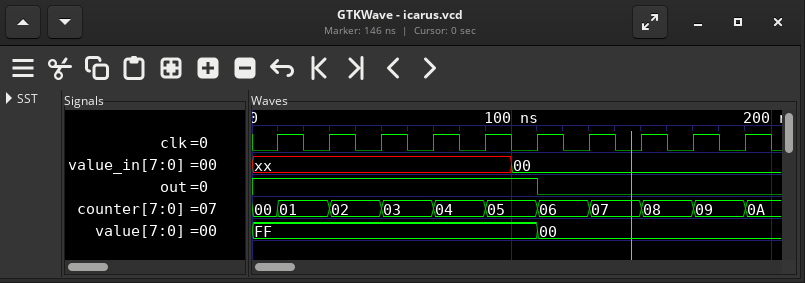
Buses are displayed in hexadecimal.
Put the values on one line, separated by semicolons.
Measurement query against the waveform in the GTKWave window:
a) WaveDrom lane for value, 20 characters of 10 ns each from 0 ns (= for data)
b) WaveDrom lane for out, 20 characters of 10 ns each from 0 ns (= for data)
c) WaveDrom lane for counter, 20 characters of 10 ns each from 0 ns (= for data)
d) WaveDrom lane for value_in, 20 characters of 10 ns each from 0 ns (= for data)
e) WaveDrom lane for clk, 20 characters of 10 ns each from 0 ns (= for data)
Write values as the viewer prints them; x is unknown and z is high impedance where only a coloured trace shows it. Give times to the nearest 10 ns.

{name: 'value', wave: '=..........=........', data: 'FF 00'}; {name: 'out', wave: '1..........0........'}; {name: 'counter', wave: '==.=.=.=.=.=.=.=.=.=', data: '00 01 02 03 04 05 06 07 08 09 0A'}; {name: 'value_in', wave: 'x.........=.........', data: '00'}; {name: 'clk', wave: '01010101010101010101'}
